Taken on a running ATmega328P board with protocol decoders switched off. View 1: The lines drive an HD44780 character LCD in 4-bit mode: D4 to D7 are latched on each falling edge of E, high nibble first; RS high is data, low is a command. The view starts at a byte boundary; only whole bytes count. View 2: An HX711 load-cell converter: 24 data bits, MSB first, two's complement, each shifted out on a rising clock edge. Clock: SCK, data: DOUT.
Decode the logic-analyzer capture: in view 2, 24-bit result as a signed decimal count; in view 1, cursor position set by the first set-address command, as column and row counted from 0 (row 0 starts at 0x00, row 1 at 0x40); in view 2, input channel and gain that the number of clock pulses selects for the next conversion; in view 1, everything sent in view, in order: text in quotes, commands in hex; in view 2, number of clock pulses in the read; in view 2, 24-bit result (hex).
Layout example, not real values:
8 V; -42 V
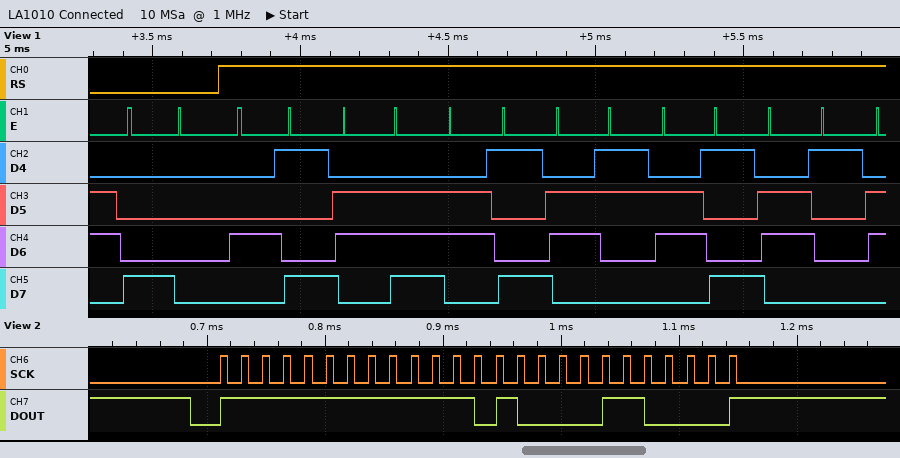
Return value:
-3024; column 0, row 0; channel A, gain 128; 0x80 "Inicia"; 25; 0xFFF430
